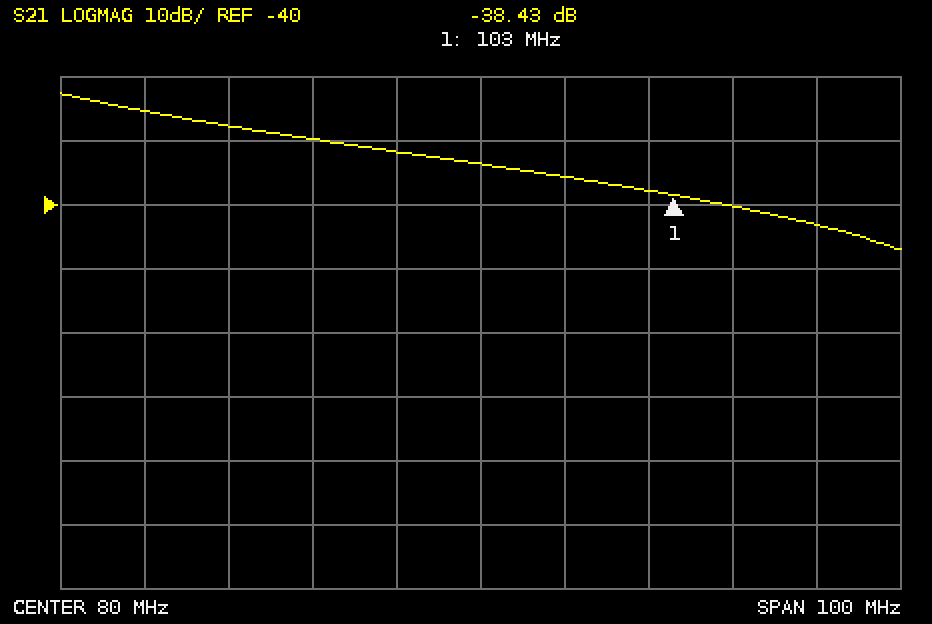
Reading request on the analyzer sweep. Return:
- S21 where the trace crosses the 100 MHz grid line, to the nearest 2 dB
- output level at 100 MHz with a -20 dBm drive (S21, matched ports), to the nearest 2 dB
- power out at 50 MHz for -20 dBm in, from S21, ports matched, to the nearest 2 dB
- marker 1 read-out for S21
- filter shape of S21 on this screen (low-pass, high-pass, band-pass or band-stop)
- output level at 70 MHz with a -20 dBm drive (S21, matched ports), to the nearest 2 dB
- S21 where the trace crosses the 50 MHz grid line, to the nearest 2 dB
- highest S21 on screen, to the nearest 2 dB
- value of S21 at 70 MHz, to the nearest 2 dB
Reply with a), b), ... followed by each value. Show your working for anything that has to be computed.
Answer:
a) -38 dB
b) -20 dBm + (-38 dB) = -58 dBm
c) -20 dBm + (-28 dB) = -48 dBm
d) -38.43 dB
e) low-pass
f) -20 dBm + (-32 dB) = -52 dBm
g) -28 dB
h) -22 dB
i) -32 dB
